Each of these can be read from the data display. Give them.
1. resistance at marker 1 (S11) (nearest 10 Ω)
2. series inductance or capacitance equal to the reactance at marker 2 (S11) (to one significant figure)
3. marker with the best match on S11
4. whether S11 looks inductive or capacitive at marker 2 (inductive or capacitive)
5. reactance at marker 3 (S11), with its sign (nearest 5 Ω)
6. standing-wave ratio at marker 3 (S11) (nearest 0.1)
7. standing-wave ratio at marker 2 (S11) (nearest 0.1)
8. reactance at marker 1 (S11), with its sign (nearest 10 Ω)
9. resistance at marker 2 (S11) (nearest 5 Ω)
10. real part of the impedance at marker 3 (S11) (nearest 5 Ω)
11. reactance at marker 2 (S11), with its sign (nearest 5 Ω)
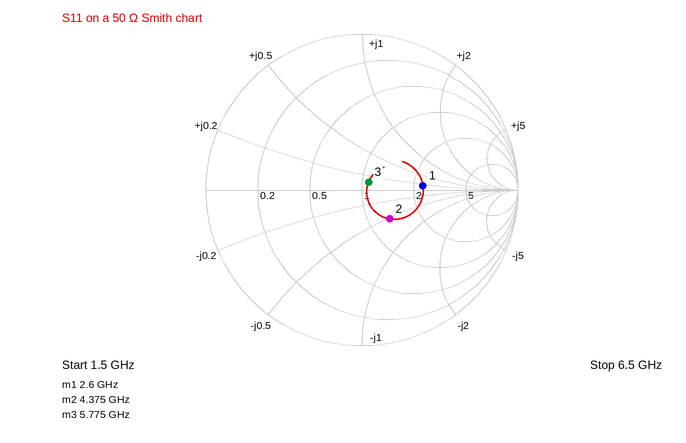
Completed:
110 Ω
1 pF
marker 3
capacitive
+5 Ω
1.1
1.7
+10 Ω
65 Ω
55 Ω
-25 Ω
